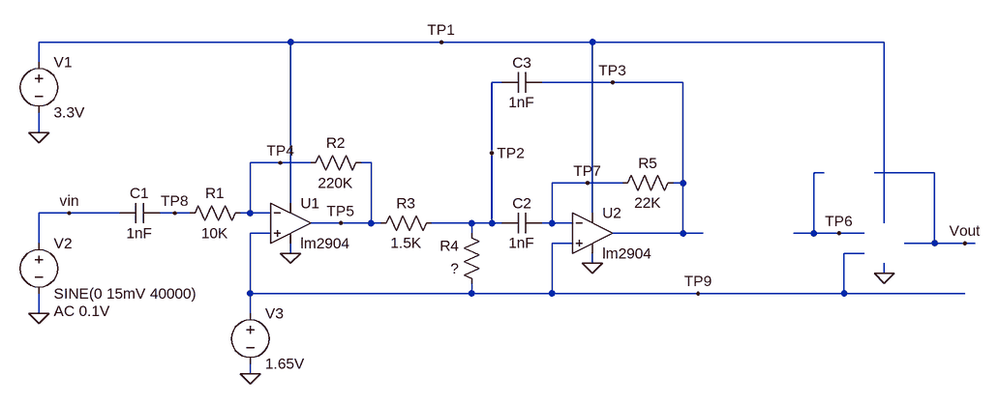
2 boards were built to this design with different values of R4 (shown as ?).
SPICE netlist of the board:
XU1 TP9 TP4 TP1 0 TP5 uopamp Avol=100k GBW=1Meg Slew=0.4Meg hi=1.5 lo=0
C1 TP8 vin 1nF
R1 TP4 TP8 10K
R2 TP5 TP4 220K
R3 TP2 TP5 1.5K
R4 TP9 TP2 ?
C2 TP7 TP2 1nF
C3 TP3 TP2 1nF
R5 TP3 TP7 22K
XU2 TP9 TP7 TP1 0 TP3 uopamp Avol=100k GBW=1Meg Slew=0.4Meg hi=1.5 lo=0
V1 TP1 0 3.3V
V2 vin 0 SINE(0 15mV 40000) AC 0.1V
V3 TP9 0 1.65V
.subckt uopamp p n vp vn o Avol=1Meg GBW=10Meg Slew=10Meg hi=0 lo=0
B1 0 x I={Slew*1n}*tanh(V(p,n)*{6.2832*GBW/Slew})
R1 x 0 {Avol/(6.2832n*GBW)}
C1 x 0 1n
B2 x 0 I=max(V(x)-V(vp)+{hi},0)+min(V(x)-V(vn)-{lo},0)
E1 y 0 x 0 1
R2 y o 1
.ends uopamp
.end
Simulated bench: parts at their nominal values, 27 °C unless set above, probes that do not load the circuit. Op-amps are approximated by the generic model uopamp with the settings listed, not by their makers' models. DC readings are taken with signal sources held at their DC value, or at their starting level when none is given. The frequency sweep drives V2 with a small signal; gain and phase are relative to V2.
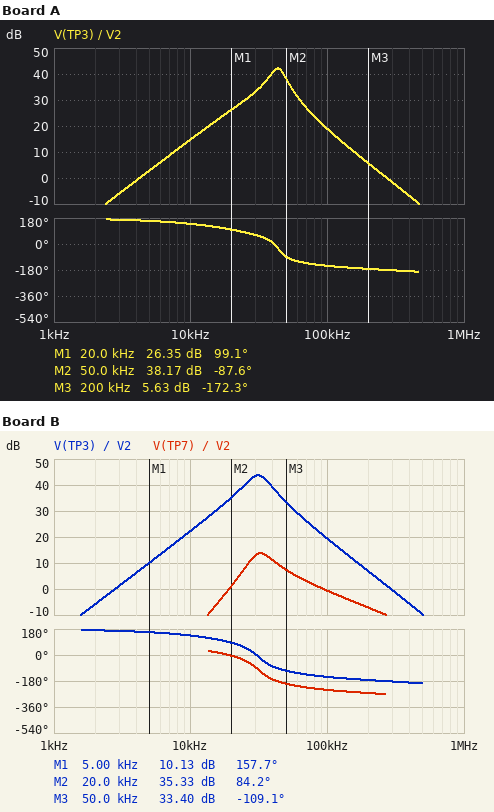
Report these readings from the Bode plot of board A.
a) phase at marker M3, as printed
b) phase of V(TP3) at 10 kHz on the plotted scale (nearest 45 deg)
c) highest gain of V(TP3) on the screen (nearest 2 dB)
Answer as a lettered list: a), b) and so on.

a) -172.3 deg
b) 135 deg
c) 42 dB
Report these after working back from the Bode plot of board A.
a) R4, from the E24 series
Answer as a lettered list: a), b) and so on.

a) 620 Ω
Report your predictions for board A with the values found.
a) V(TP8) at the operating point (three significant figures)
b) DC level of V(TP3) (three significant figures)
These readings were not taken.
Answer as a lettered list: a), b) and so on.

a) 1.65 V
b) 1.65 V
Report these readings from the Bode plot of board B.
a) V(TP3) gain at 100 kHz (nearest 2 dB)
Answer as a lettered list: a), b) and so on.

a) 20 dB
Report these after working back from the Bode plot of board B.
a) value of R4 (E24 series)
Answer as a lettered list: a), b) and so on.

a) 3 kΩ
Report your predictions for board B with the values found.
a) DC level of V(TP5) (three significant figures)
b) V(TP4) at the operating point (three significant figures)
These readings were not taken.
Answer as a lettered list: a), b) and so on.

a) 1.65 V
b) 1.65 V
